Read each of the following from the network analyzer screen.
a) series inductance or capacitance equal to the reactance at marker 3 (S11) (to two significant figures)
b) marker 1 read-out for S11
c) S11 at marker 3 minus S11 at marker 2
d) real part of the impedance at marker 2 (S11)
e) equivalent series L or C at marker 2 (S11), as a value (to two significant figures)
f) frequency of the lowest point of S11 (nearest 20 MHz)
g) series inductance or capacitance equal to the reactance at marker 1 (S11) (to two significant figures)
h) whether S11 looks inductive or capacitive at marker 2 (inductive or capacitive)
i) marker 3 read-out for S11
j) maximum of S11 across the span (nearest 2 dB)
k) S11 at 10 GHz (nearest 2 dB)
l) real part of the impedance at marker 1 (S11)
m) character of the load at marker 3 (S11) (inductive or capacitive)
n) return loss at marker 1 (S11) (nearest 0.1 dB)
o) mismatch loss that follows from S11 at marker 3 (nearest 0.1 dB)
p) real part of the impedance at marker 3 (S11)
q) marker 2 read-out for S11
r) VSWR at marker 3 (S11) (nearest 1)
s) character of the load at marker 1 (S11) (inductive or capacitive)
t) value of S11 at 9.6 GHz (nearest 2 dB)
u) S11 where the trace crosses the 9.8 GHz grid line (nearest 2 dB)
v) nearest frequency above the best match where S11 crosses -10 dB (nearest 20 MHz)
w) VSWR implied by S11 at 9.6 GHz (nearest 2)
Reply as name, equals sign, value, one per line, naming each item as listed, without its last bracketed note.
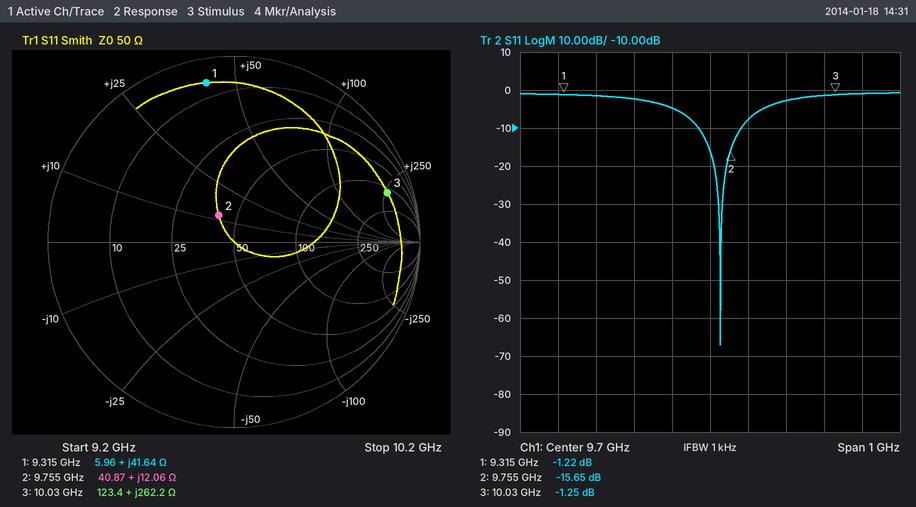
series inductance or capacitance equal to the reactance at marker 3 (S11) = 4.2 nH
marker 1 read-out for S11 = -1.22 dB
S11 at marker 3 minus S11 at marker 2 = 14.40 dB
real part of the impedance at marker 2 = 40.87 Ω
equivalent series L or C at marker 2 (S11), as a value = 200 pH
frequency of the lowest point of S11 = 9.72 GHz
series inductance or capacitance equal to the reactance at marker 1 (S11) = 710 pH
whether S11 looks inductive or capacitive at marker 2 = inductive
marker 3 read-out for S11 = -1.25 dB
maximum of S11 across the span = 0 dB
S11 at 10 GHz = -2 dB
real part of the impedance at marker 1 = 5.96 Ω
character of the load at marker 3 (S11) = inductive
return loss at marker 1 (S11) = 1.2 dB
mismatch loss that follows from S11 at marker 3 = 6.0 dB
real part of the impedance at marker 3 = 123.4 Ω
marker 2 read-out for S11 = -15.65 dB
VSWR at marker 3 (S11) = 14
character of the load at marker 1 (S11) = inductive
value of S11 at 9.6 GHz = -4 dB
S11 where the trace crosses the 9.8 GHz grid line = -8 dB
nearest frequency above the best match where S11 crosses -10 dB = 9.78 GHz
VSWR implied by S11 at 9.6 GHz = 4
